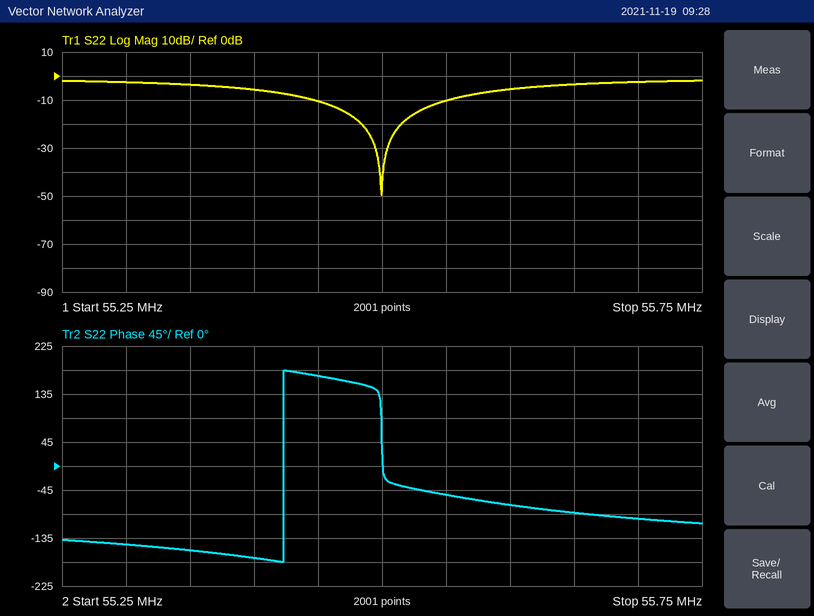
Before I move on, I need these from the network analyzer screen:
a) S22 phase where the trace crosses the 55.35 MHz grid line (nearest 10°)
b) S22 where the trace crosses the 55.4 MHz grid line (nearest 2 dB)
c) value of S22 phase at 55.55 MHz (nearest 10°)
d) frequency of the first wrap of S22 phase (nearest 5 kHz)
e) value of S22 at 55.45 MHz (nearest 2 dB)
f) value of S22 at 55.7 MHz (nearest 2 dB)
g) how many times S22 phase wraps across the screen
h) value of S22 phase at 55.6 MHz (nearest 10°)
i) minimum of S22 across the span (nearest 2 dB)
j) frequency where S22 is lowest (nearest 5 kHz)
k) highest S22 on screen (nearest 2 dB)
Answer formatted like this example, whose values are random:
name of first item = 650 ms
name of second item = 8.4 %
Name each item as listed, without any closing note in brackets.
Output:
S22 phase where the trace crosses the 55.35 MHz grid line = -160°
S22 where the trace crosses the 55.4 MHz grid line = -6 dB
value of S22 phase at 55.55 MHz = -50°
frequency of the first wrap of S22 phase = 55.425 MHz
value of S22 at 55.45 MHz = -10 dB
value of S22 at 55.7 MHz = -2 dB
how many times S22 phase wraps across the screen = 1
value of S22 phase at 55.6 MHz = -70°
minimum of S22 across the span = -50 dB
frequency where S22 is lowest = 55.500 MHz
highest S22 on screen = -2 dB
